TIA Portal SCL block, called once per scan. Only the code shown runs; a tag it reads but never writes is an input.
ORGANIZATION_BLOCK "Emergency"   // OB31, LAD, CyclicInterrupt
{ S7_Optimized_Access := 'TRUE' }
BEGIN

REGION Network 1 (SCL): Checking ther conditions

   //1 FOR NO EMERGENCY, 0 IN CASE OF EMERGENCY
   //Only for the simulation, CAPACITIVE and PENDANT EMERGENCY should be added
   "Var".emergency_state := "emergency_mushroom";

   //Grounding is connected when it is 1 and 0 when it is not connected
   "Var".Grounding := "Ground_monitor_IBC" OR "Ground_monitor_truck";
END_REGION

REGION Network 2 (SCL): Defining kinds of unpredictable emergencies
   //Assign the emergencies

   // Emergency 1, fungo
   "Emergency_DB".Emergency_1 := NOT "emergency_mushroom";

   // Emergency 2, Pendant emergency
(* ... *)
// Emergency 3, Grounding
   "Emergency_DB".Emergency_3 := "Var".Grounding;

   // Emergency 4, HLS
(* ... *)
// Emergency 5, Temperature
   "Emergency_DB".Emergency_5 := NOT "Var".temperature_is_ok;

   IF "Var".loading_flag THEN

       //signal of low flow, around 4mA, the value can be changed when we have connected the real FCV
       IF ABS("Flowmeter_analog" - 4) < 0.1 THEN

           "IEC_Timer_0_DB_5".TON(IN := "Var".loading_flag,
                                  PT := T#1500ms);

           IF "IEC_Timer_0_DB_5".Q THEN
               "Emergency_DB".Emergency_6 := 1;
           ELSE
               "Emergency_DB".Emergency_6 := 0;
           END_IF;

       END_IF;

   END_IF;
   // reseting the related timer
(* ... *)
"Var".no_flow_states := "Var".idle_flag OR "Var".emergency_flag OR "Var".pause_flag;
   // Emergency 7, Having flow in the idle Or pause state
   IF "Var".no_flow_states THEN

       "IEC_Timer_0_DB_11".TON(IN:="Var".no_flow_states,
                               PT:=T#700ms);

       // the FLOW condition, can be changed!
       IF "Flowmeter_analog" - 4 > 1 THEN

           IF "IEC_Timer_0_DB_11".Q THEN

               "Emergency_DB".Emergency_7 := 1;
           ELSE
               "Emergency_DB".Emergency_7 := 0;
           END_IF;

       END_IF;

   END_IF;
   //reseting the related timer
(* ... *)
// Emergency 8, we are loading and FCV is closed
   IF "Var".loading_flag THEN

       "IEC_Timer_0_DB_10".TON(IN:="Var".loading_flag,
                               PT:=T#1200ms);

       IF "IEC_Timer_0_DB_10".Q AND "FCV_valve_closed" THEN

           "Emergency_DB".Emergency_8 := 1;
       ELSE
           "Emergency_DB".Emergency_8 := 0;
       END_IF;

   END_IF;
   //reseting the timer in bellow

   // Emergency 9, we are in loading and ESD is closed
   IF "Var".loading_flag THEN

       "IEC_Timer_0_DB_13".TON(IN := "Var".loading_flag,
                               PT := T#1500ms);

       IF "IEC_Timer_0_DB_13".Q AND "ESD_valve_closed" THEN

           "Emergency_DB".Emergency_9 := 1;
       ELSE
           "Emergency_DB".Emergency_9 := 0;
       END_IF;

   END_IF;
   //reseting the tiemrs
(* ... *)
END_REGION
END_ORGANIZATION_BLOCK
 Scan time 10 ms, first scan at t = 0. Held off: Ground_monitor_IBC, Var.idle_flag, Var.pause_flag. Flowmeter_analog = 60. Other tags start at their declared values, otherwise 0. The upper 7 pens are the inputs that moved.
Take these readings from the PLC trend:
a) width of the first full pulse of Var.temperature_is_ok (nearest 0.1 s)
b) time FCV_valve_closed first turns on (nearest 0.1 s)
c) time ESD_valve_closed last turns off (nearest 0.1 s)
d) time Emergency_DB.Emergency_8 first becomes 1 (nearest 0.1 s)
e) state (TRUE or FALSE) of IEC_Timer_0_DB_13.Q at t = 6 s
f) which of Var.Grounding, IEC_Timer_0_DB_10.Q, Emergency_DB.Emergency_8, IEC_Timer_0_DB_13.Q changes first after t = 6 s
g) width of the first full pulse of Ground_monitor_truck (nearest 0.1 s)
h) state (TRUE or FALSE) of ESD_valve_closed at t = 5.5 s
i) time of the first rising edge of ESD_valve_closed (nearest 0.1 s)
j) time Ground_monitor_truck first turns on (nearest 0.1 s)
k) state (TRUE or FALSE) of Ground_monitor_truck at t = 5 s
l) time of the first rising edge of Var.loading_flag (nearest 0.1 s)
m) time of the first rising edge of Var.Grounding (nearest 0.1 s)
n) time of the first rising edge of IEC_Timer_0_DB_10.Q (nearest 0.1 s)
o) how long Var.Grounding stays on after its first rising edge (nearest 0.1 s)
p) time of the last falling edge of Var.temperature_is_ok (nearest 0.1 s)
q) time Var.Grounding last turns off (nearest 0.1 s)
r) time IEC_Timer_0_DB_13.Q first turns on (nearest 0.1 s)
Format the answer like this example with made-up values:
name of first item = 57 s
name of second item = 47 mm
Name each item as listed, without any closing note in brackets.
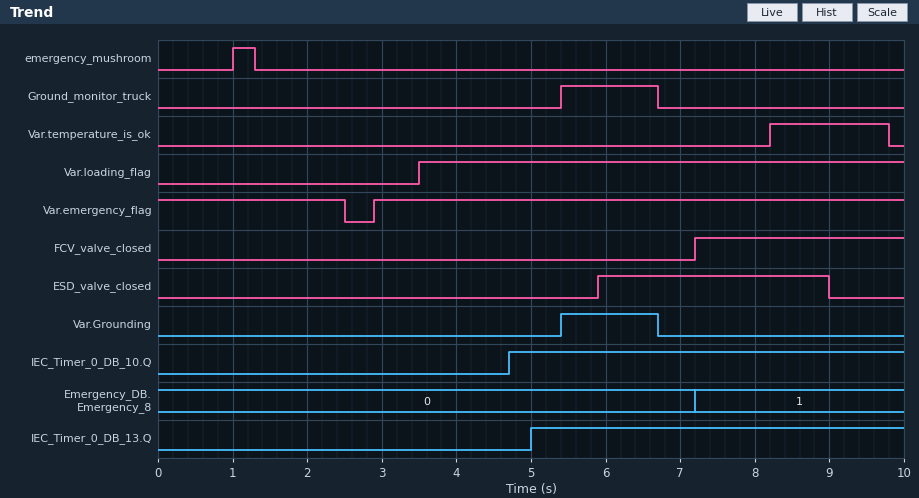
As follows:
width of the first full pulse of Var.temperature_is_ok = 1.6 s
time FCV_valve_closed first turns on = 7.2 s
time ESD_valve_closed last turns off = 9.0 s
time Emergency_DB.Emergency_8 first becomes 1 = 7.2 s
state (TRUE or FALSE) of IEC_Timer_0_DB_13.Q at t = 6 s = TRUE
which of Var.Grounding, IEC_Timer_0_DB_10.Q, Emergency_DB.Emergency_8, IEC_Timer_0_DB_13.Q changes first after t = 6 s = Var.Grounding
width of the first full pulse of Ground_monitor_truck = 1.3 s
state (TRUE or FALSE) of ESD_valve_closed at t = 5.5 s = FALSE
time of the first rising edge of ESD_valve_closed = 5.9 s
time Ground_monitor_truck first turns on = 5.4 s
state (TRUE or FALSE) of Ground_monitor_truck at t = 5 s = FALSE
time of the first rising edge of Var.loading_flag = 3.5 s
time of the first rising edge of Var.Grounding = 5.4 s
time of the first rising edge of IEC_Timer_0_DB_10.Q = 4.7 s
how long Var.Grounding stays on after its first rising edge = 1.3 s
time of the last falling edge of Var.temperature_is_ok = 9.8 s
time Var.Grounding last turns off = 6.7 s
time IEC_Timer_0_DB_13.Q first turns on = 5.0 s
